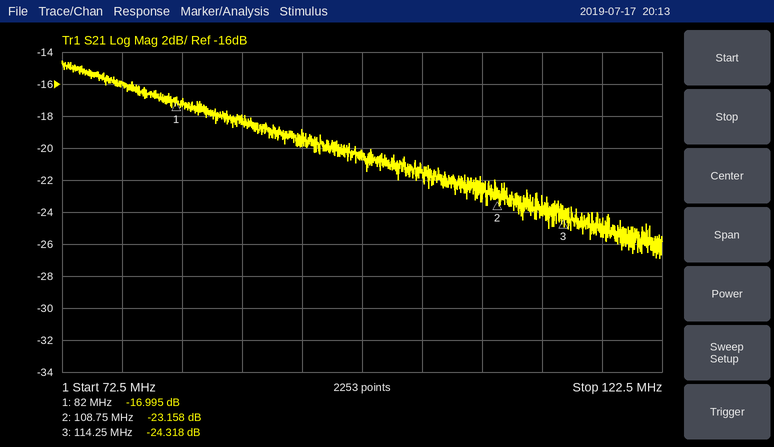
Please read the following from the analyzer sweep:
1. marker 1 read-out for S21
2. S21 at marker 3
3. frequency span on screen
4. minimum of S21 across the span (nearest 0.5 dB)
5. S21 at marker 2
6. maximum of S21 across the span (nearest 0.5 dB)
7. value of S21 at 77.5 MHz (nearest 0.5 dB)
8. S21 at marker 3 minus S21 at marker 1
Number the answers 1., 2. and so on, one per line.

1. -16.995 dB
2. -24.318 dB
3. 50 MHz
4. -27.0 dB
5. -23.158 dB
6. -14.5 dB
7. -16.0 dB
8. -7.323 dB
